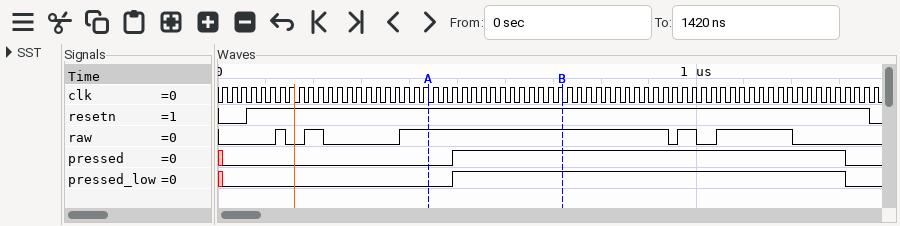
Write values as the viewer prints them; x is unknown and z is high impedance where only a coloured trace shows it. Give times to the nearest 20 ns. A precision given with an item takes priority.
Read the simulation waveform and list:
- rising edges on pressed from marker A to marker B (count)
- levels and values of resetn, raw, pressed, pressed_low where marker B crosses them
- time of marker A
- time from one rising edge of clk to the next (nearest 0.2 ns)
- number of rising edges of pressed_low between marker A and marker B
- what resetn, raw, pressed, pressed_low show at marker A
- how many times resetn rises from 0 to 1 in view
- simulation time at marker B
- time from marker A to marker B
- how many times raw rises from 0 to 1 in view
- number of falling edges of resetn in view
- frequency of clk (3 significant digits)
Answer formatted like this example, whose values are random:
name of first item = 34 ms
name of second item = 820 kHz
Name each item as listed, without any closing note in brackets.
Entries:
rising edges on pressed from marker A to marker B = 1
levels and values of resetn, raw, pressed, pressed_low where marker B crosses them = resetn=1, raw=1, pressed=1, pressed_low=1
time of marker A = 440 ns
time from one rising edge of clk to the next = 20 ns
number of rising edges of pressed_low between marker A and marker B = 1
what resetn, raw, pressed, pressed_low show at marker A = resetn=1, raw=1, pressed=0, pressed_low=0
how many times resetn rises from 0 to 1 in view = 1
simulation time at marker B = 720 ns
time from marker A to marker B = 280 ns
how many times raw rises from 0 to 1 in view = 5
number of falling edges of resetn in view = 1
frequency of clk = 50.0 MHz
